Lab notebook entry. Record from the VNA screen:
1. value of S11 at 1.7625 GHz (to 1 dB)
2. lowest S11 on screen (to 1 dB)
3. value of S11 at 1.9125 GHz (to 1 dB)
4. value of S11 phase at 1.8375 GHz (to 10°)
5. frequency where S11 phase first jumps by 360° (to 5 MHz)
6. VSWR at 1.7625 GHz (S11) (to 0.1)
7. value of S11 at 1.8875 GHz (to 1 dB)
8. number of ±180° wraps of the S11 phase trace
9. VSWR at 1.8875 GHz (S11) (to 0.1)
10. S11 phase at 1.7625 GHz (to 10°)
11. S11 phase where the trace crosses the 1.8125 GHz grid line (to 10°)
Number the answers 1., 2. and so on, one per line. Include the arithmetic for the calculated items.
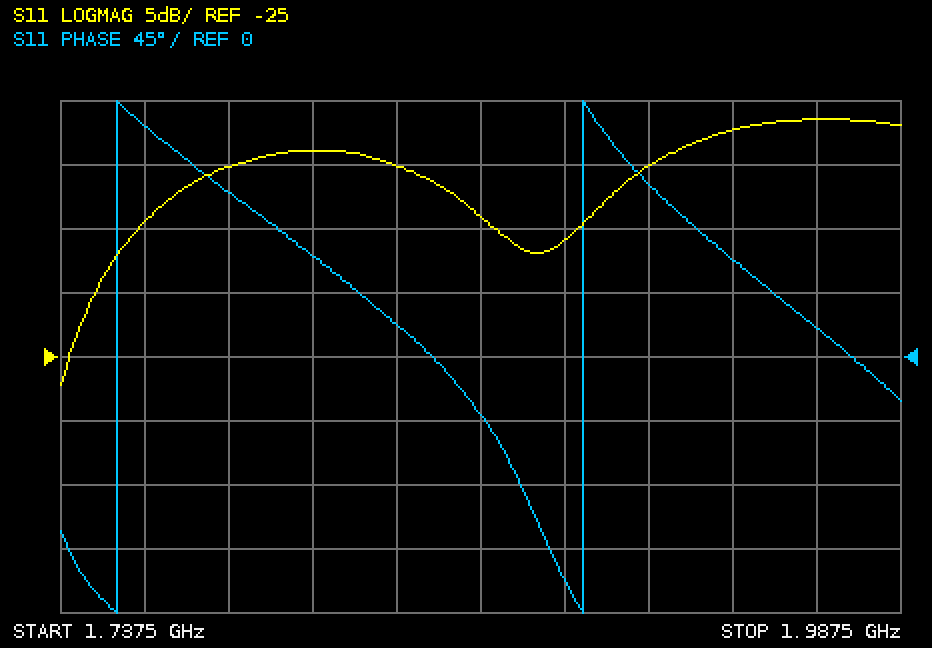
1. -14 dB
2. -27 dB
3. -10 dB
4. 20°
5. 1.755 GHz
6. |Γ| = 10^(-14/20) = 0.1995; VSWR = (1 + 0.1995)/(1 − 0.1995) ≈ 1.5
7. -16 dB
8. 2
9. |Γ| = 10^(-16/20) = 0.1585; VSWR = (1 + 0.1585)/(1 − 0.1585) ≈ 1.4
10. 160°
11. 70°
